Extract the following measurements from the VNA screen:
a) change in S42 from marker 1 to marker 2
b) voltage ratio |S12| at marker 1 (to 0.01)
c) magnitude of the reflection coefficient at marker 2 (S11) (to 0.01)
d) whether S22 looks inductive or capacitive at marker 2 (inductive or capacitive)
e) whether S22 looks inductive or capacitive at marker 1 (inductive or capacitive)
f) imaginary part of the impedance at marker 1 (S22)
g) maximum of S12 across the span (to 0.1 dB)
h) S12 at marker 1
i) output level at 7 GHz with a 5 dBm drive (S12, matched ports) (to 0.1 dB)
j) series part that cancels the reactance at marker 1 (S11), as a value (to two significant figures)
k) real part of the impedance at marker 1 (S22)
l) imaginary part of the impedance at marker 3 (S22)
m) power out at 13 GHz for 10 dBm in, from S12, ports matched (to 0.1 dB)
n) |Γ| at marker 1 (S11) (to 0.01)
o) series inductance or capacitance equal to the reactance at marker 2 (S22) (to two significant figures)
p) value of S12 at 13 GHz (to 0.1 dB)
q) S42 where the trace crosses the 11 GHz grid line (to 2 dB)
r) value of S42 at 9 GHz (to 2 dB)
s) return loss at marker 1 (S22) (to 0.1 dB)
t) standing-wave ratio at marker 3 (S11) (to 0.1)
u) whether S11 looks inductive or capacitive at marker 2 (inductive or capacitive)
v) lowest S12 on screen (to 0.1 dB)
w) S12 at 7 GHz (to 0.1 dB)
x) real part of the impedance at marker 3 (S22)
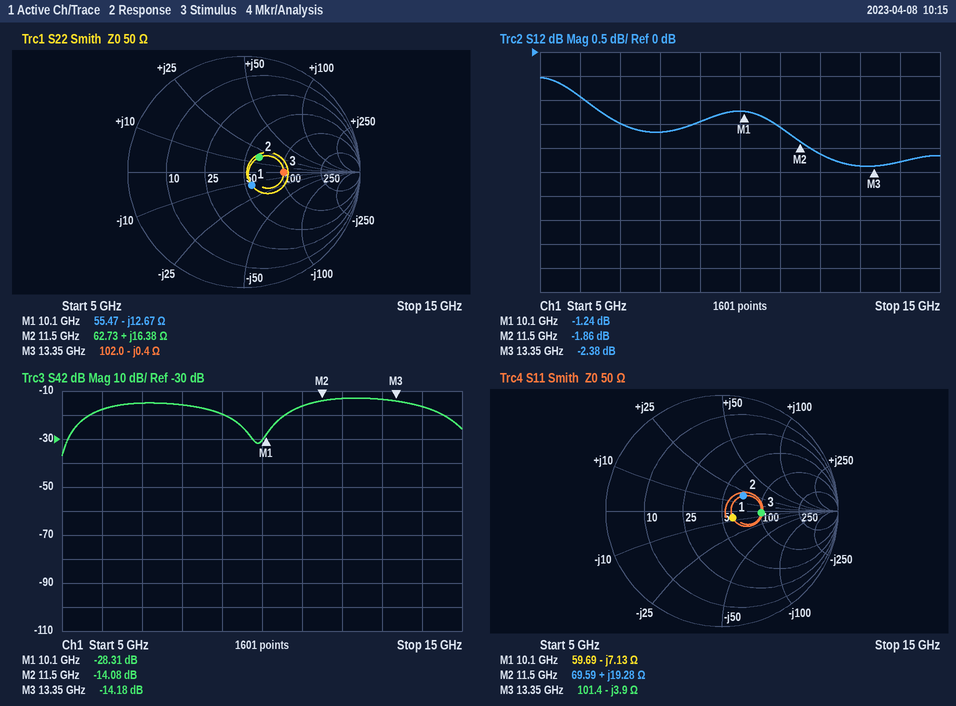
14.23 dB
0.87
0.23
inductive
capacitive
-12.67 Ω
-0.5 dB
-1.24 dB
3.5 dBm
110 pH
55.47 Ω
-0.4 Ω
7.6 dBm
0.11
230 pH
-2.4 dB
-16 dB
-20 dB
17.7 dB
2.0
inductive
-2.4 dB
-1.5 dB
102.0 Ω
